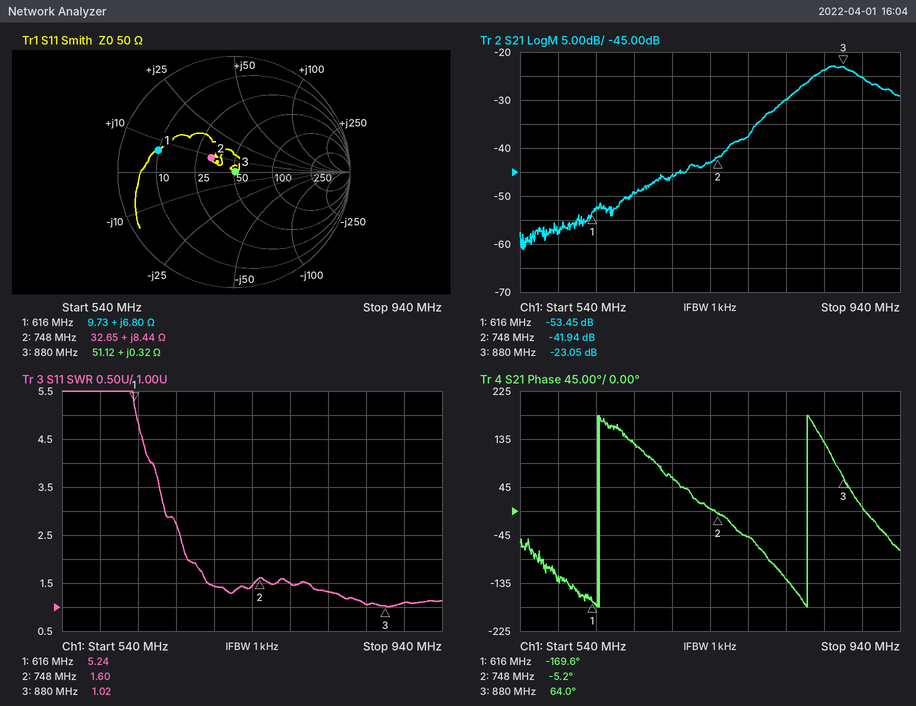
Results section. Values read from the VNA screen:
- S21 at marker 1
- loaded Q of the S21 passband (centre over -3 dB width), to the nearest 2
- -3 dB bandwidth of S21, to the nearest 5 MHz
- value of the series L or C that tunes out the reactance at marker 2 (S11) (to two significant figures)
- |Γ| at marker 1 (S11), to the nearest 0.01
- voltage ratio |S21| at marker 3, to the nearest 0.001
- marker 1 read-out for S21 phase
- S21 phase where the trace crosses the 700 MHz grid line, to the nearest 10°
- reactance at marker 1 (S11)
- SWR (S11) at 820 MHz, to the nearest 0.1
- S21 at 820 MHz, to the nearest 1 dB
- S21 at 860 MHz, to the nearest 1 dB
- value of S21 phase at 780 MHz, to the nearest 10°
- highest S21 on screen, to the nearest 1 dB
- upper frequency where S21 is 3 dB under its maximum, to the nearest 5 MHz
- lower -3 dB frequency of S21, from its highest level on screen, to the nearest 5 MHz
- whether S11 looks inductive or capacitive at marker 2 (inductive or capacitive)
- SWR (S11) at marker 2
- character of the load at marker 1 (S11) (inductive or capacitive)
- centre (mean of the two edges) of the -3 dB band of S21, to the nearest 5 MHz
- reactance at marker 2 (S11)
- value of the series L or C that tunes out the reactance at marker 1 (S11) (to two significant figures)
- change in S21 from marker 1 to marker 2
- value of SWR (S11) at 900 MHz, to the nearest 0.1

-53.45 dB
14
60 MHz
25 pF
0.68
0.070
-169.6°
60°
+6.80 Ω
1.3
-30 dB
-24 dB
-50°
-23 dB
905 MHz
845 MHz
inductive
1.60
inductive
875 MHz
+8.44 Ω
38 pF
11.51 dB
1.1
